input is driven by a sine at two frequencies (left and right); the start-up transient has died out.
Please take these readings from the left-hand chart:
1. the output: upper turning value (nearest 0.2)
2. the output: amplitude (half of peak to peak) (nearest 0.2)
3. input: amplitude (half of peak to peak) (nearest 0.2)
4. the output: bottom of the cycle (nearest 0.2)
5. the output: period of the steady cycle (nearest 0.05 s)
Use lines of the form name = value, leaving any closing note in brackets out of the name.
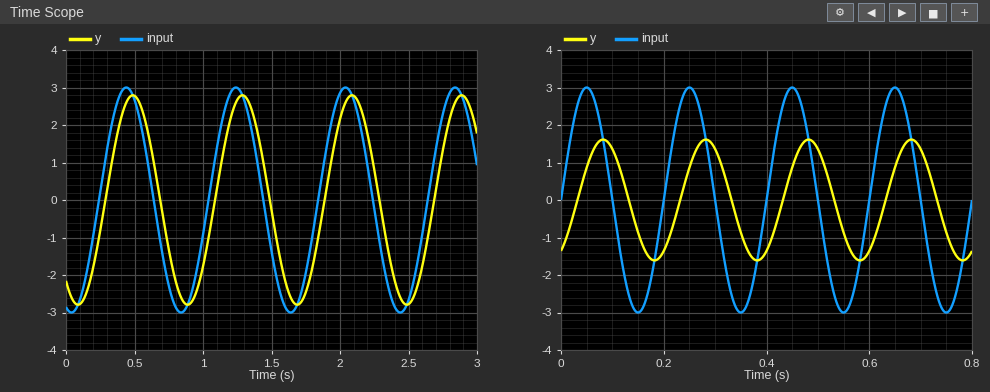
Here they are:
the output: upper turning value = 2.8
the output: amplitude (half of peak to peak) = 2.8
input: amplitude (half of peak to peak) = 3.0
the output: bottom of the cycle = -2.8
the output: period of the steady cycle = 0.80 s
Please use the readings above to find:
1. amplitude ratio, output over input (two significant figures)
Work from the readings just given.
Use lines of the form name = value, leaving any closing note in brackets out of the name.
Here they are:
amplitude ratio, output over input = 0.93
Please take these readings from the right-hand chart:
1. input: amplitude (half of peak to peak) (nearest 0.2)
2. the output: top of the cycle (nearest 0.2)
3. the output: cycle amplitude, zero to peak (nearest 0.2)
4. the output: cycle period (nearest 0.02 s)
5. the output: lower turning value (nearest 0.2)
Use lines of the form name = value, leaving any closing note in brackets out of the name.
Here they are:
input: amplitude (half of peak to peak) = 3.0
the output: top of the cycle = 1.6
the output: cycle amplitude, zero to peak = 1.6
the output: cycle period = 0.20 s
the output: lower turning value = -1.6
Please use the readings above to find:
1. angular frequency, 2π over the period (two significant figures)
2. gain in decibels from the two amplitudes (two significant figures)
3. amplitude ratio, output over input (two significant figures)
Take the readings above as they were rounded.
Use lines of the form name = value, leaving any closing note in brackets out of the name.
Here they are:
angular frequency, 2π over the period = 31 rad/s
gain in decibels from the two amplitudes = -5.5 dB
amplitude ratio, output over input = 0.53
